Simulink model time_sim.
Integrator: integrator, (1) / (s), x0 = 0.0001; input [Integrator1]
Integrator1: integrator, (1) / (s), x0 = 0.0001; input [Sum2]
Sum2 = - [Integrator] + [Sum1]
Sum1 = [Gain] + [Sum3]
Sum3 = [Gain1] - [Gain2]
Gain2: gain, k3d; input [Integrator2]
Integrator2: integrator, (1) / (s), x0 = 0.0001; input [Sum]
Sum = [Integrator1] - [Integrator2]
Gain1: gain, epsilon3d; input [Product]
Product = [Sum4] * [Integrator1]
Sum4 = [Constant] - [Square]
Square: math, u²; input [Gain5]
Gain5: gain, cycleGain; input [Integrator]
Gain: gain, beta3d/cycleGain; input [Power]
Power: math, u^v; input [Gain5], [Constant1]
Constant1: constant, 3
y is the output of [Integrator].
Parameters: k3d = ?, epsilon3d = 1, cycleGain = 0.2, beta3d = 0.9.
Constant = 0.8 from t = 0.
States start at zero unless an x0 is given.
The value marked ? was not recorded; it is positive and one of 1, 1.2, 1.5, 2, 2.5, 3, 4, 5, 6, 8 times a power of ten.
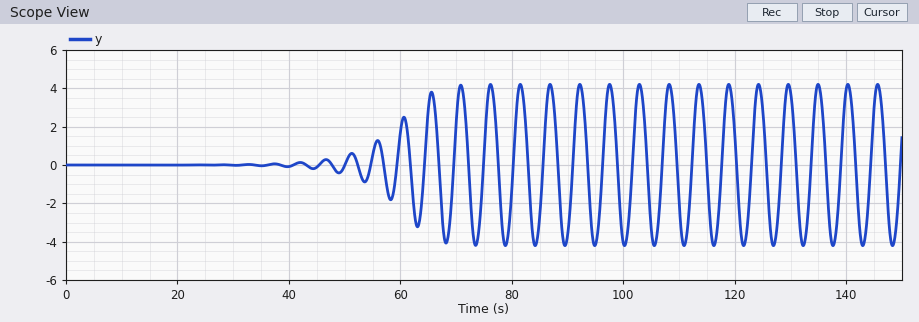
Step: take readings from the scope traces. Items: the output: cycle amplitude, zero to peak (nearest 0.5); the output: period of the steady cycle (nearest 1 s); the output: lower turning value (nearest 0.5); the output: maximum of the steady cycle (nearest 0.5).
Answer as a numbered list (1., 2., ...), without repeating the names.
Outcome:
1. 4.0
2. 5 s
3. -4.0
4. 4.0
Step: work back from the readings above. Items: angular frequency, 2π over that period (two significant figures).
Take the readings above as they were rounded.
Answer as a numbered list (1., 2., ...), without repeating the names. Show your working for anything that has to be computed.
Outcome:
1. 2π / 5 = 1.3 rad/s
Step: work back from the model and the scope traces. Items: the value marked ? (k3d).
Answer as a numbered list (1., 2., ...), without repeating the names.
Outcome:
1. 1.5
